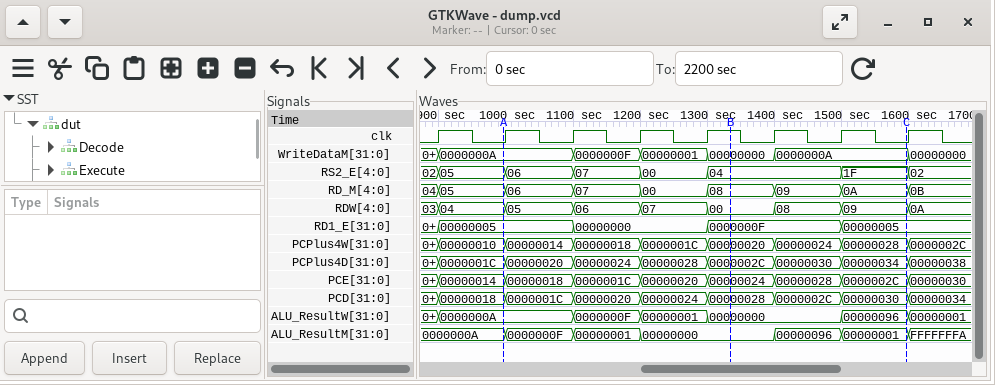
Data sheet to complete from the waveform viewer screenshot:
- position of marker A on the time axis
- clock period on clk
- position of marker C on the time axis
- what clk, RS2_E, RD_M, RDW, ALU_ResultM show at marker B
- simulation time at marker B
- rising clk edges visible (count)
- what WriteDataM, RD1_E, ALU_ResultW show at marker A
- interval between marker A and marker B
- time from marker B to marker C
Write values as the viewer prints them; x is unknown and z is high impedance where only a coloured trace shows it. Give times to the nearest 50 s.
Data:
1000 s
100 s
1600 s
clk=1, RS2_E=04, RD_M=08, RDW=00, ALU_ResultM=00000000
1350 s
8
WriteDataM=0000000A, RD1_E=00000005, ALU_ResultW=0000000A
350 s
250 s
